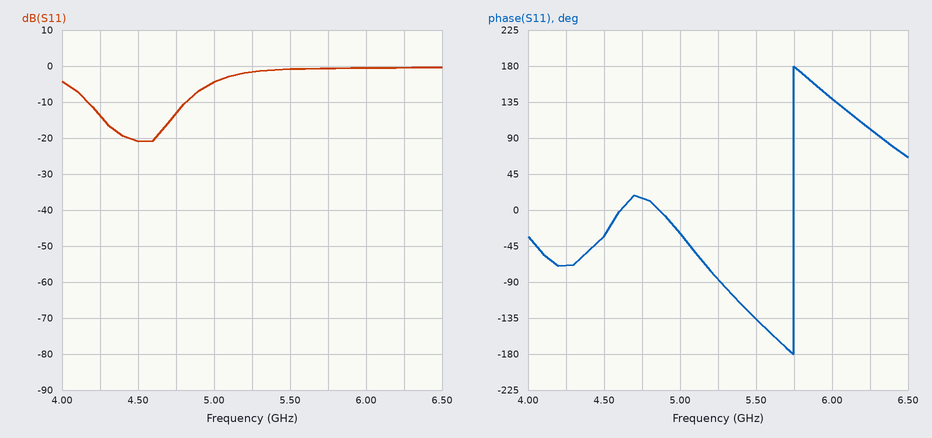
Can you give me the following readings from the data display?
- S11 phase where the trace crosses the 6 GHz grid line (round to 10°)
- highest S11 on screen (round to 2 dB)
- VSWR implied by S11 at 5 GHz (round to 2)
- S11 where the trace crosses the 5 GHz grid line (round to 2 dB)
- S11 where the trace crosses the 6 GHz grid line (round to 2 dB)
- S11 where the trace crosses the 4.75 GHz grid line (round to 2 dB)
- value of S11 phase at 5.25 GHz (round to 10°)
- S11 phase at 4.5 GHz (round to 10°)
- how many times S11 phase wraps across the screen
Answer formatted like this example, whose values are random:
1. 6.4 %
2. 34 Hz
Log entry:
1. 140°
2. 0 dB
3. 4
4. -4 dB
5. 0 dB
6. -14 dB
7. -90°
8. -30°
9. 1
